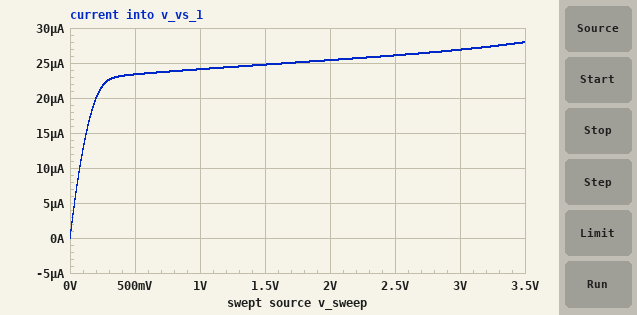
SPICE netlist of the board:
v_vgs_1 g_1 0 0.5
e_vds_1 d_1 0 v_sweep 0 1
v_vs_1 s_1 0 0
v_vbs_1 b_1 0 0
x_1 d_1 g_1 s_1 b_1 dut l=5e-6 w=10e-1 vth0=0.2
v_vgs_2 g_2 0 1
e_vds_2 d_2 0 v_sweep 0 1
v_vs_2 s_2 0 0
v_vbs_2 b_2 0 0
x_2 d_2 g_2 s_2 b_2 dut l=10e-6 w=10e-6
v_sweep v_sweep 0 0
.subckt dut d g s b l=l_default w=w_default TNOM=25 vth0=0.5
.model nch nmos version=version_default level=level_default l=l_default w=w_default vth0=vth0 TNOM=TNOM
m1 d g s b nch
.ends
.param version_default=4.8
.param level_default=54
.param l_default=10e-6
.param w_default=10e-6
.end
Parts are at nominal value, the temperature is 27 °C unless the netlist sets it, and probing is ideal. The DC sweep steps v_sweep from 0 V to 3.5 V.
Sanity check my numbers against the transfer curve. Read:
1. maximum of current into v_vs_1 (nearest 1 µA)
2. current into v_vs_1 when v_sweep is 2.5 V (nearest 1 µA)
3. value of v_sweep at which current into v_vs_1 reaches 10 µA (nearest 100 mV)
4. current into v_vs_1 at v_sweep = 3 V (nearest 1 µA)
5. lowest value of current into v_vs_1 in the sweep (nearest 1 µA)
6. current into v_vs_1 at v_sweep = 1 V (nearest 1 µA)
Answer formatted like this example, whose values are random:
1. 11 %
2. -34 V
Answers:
1. 28 µA
2. 26 µA
3. 100 mV
4. 27 µA
5. 0 A
6. 24 µA
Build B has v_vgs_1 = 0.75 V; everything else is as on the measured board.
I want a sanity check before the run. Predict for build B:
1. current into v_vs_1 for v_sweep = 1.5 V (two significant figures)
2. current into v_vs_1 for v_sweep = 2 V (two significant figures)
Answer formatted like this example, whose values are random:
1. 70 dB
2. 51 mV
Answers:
1. 75 µA
2. 76 µA
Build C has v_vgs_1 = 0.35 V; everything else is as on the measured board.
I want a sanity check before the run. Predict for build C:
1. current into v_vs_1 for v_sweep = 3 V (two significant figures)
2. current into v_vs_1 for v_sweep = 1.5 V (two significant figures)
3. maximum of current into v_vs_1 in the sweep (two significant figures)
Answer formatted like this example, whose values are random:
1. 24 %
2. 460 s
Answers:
1. 7.3 µA
2. 6.4 µA
3. 7.7 µA
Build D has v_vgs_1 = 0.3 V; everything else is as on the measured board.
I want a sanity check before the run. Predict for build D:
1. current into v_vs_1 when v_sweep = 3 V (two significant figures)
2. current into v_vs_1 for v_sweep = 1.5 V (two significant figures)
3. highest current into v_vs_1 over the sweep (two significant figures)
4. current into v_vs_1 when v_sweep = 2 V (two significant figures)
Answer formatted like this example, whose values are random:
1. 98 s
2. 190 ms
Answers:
1. 3.5 µA
2. 2.9 µA
3. 3.7 µA
4. 3.1 µA
